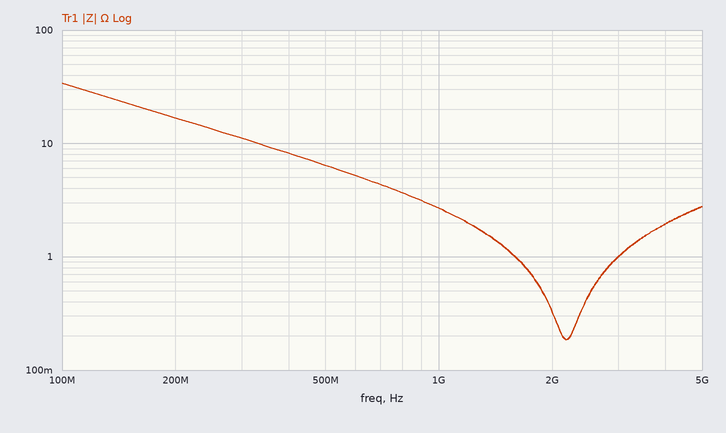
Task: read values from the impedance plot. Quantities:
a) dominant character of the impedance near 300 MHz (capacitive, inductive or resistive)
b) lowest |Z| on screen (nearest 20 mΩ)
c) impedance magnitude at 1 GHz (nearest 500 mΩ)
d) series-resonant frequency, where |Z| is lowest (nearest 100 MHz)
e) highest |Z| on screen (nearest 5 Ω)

capacitive
180 mΩ
2.5 Ω
2.2 GHz
35 Ω
